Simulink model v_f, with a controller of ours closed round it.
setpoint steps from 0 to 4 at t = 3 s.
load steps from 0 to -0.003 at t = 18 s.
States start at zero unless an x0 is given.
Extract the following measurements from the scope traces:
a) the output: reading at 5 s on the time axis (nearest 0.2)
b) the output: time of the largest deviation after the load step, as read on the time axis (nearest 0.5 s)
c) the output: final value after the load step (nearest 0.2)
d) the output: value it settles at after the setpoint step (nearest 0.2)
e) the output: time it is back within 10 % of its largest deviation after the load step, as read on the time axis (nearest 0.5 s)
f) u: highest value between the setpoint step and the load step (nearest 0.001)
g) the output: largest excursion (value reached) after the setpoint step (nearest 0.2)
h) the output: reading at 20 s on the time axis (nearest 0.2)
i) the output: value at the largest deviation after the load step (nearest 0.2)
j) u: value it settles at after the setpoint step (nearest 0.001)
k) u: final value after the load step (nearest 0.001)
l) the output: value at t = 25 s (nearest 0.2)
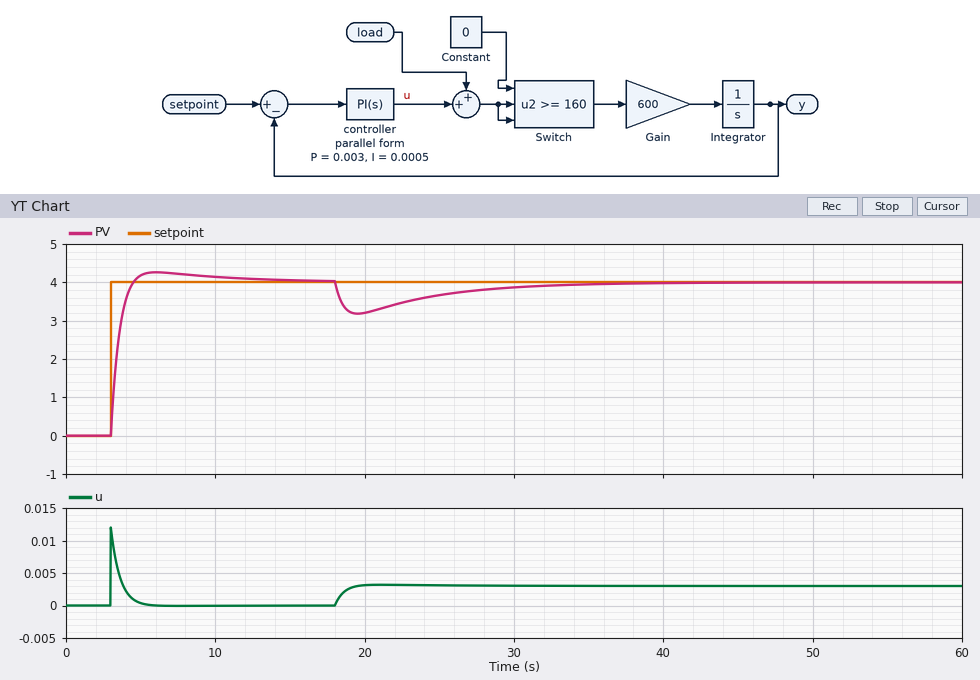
4.2
19.5 s
4.0
4.0
32.5 s
0.012
4.2
3.2
3.2
0.000
0.003
3.6
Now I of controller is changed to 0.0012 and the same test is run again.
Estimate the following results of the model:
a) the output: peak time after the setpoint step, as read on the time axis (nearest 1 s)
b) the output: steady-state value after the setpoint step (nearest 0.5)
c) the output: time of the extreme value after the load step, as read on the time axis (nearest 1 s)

5 s
4.0
19 s
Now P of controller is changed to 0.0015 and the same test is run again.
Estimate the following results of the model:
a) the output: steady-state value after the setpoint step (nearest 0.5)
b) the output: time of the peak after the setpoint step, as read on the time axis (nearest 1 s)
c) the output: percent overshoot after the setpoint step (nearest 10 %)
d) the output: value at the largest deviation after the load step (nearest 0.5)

4.0
7 s
20 %
2.5
